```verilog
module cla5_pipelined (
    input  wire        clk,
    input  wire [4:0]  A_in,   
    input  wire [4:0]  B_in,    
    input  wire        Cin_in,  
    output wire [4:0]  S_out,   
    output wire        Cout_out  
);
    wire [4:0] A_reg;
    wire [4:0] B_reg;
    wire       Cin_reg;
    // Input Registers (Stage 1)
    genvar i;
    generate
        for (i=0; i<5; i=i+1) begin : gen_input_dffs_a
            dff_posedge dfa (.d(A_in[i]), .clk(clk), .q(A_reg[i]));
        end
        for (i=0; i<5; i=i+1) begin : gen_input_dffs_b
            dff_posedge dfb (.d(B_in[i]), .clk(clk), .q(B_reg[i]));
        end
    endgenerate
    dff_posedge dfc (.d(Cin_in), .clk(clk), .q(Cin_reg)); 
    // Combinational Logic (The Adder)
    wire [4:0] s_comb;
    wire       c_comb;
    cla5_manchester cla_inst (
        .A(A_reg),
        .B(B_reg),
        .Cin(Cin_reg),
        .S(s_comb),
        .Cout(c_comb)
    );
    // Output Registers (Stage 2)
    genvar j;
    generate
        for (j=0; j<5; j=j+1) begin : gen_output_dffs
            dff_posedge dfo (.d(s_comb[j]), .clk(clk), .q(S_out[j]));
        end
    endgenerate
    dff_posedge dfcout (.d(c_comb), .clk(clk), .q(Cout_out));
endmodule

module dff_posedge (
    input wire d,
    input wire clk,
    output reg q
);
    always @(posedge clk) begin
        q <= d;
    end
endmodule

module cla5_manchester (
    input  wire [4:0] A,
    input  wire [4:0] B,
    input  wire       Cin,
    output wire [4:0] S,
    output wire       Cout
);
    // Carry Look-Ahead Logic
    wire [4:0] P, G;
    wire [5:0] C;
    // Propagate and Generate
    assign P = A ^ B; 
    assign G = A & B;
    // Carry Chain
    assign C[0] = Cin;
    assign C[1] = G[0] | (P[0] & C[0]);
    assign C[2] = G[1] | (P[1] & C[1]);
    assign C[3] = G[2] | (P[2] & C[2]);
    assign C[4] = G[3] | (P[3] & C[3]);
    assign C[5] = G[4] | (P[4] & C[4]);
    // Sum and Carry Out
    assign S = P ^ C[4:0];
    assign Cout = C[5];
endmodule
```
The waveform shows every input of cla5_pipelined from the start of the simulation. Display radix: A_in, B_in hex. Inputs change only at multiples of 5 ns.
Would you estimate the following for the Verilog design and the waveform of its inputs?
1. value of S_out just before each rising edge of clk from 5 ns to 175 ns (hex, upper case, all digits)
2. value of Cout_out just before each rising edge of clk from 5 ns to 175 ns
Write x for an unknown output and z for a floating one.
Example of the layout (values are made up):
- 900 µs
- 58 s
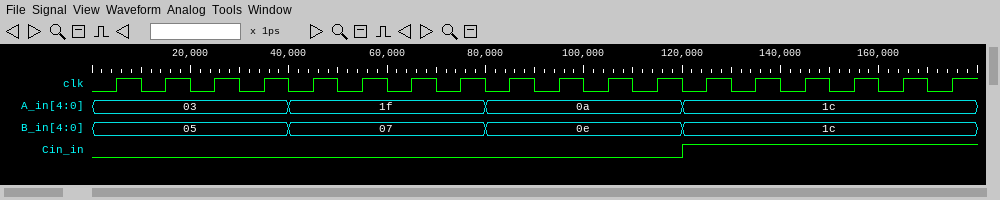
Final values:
- x, x, 08, 08, 08, 08, 06, 06, 06, 06, 18, 18, 18, 18, 19, 19, 19, 19
- x x 0 0 0 0 1 1 1 1 0 0 0 0 1 1 1 1
